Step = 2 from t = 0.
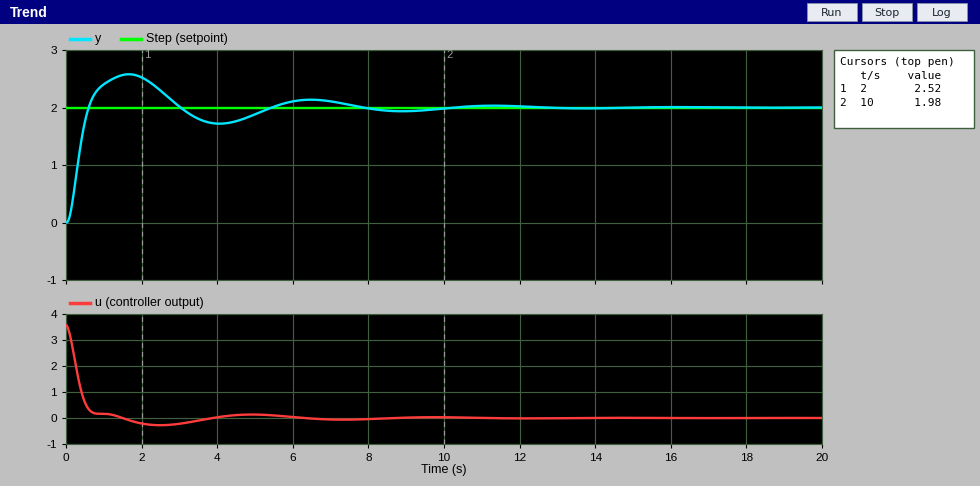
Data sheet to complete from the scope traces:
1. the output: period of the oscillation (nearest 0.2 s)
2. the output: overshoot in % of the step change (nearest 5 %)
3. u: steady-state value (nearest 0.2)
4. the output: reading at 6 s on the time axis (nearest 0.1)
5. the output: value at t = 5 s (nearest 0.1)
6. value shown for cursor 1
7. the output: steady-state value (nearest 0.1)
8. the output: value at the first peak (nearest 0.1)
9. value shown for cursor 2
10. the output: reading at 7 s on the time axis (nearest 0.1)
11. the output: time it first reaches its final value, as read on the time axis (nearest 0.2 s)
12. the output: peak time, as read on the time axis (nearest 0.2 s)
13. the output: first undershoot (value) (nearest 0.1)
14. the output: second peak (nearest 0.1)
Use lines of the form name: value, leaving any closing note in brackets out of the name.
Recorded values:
the output: period of the oscillation: 4.8 s
the output: overshoot in % of the step change: 30 %
u: steady-state value: 0.0
the output: reading at 6 s on the time axis: 2.1
the output: value at t = 5 s: 1.9
value shown for cursor 1: 2.52
the output: steady-state value: 2.0
the output: value at the first peak: 2.6
value shown for cursor 2: 1.98
the output: reading at 7 s on the time axis: 2.1
the output: time it first reaches its final value, as read on the time axis: 0.6 s
the output: peak time, as read on the time axis: 1.6 s
the output: first undershoot (value): 1.7
the output: second peak: 2.1
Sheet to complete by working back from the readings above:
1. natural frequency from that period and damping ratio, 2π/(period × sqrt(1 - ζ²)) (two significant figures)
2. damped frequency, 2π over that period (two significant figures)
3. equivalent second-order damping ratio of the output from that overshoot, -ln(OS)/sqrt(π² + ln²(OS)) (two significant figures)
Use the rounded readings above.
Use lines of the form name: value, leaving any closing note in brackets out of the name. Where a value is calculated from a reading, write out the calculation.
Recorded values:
natural frequency from that period and damping ratio, 2π/(period × sqrt(1 - ζ²)): 2π / (4.8 × sqrt(1 - 0.36²)) = 1.4 rad/s
damped frequency, 2π over that period: 2π / 4.8 = 1.3 rad/s
equivalent second-order damping ratio of the output from that overshoot, -ln(OS)/sqrt(π² + ln²(OS)): ln(0.3) = -1.204; 1.204 / sqrt(9.870 + 1.450) = 0.36
